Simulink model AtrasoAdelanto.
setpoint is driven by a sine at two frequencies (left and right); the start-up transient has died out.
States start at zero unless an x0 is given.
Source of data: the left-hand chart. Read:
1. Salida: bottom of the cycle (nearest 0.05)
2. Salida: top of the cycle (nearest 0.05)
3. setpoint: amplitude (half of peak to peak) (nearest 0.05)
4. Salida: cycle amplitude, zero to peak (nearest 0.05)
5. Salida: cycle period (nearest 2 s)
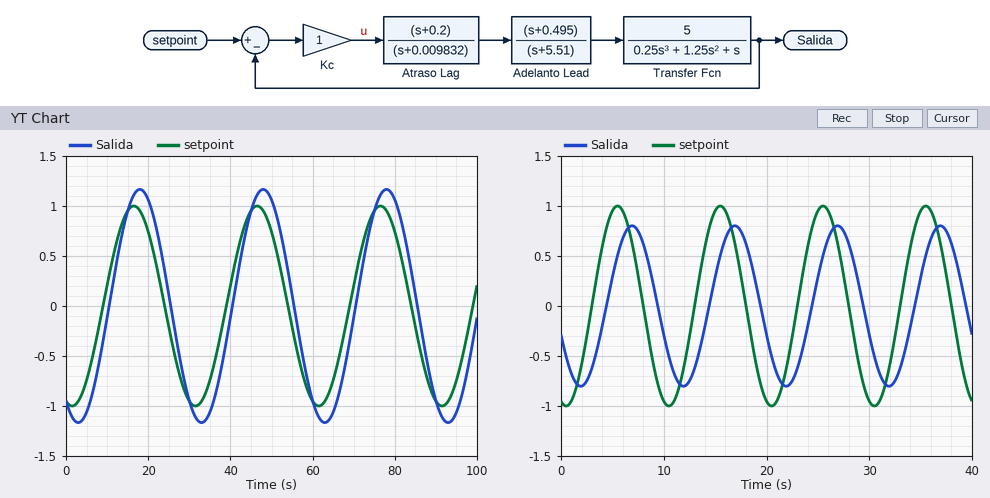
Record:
-1.15
1.15
1.00
1.15
30 s
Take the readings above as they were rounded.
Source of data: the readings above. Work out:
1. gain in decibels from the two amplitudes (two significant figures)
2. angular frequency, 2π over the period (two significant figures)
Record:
1.2 dB
0.21 rad/s
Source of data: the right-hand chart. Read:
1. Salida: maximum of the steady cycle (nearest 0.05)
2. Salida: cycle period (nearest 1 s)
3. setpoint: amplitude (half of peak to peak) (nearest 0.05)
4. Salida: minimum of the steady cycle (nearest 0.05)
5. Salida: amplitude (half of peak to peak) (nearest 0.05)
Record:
0.80
10 s
1.00
-0.80
0.80
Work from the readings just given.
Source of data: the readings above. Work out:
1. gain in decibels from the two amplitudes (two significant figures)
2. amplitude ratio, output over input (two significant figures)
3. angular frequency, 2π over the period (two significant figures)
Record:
-1.9 dB
0.80
0.63 rad/s
